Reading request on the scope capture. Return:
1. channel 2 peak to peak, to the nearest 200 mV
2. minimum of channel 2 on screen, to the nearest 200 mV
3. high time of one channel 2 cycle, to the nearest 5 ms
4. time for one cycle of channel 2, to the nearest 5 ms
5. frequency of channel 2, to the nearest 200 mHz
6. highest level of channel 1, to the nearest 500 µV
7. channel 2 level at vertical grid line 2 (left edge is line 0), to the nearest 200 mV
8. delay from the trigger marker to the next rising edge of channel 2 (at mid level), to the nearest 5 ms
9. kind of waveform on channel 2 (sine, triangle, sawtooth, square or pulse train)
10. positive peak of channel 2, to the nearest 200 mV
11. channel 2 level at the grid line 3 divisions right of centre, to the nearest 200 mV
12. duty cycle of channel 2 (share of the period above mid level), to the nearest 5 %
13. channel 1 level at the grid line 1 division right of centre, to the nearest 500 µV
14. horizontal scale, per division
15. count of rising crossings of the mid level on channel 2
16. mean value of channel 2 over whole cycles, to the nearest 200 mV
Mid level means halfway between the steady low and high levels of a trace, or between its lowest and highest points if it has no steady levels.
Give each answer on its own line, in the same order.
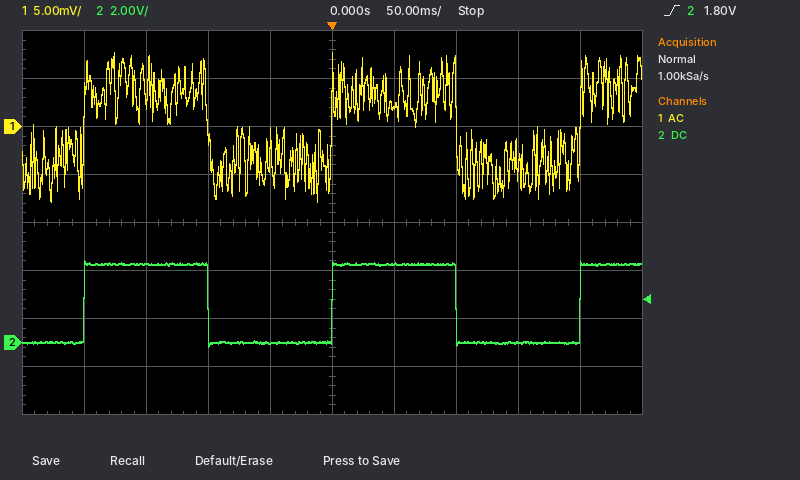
3.6 V
-200 mV
100 ms
200 ms
5.0 Hz
7.5 mV
3.2 V
200 ms
square
3.4 V
0.0 V
50 %
2.0 mV
50 ms
3
1.6 V
